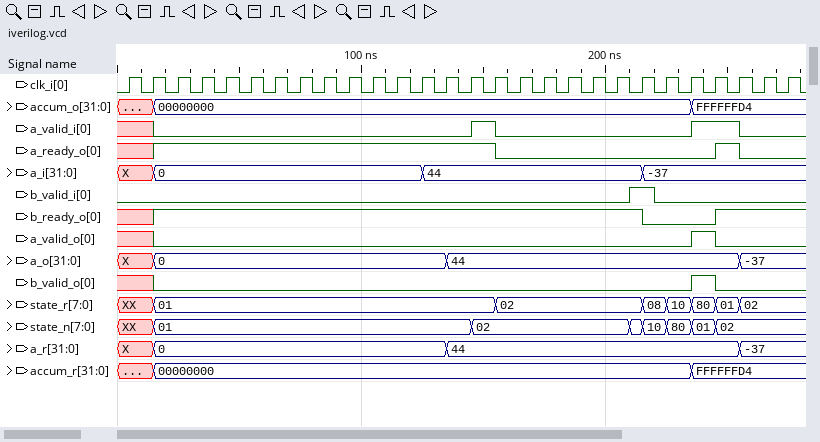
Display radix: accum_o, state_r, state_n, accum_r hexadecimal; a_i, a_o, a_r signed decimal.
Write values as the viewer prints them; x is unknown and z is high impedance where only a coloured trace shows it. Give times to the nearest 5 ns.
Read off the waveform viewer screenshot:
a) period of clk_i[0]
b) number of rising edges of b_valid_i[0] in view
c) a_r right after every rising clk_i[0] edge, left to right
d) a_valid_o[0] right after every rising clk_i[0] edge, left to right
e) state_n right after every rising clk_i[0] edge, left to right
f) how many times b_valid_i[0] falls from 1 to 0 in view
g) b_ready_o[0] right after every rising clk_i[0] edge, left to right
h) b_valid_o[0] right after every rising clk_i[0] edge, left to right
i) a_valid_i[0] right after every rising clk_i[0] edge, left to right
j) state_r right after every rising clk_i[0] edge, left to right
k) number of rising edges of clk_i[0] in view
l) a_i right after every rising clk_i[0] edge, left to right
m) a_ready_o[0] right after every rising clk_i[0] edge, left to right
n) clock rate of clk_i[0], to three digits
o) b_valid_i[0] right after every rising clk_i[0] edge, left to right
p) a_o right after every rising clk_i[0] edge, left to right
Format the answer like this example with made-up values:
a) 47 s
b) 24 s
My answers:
a) 10 ns
b) 1
c) X, 0, 0, 0, 0, 0, 0, 0, 0, 0, 0, 0, 0, 44, 44, 44, 44, 44, 44, 44, 44, 44, 44, 44, 44, -37, -37, -37
d) x 0 0 0 0 0 0 0 0 0 0 0 0 0 0 0 0 0 0 0 0 0 0 1 0 0 0 0
e) XX, 01, 01, 01, 01, 01, 01, 01, 01, 01, 01, 01, 01, 01, 02, 02, 02, 02, 02, 02, 02, 10, 80, 01, 02, 02, 02, 02
f) 1
g) x 1 1 1 1 1 1 1 1 1 1 1 1 1 1 1 1 1 1 1 1 0 0 0 1 1 1 1
h) x 0 0 0 0 0 0 0 0 0 0 0 0 0 0 0 0 0 0 0 0 0 0 1 0 0 0 0
i) x 0 0 0 0 0 0 0 0 0 0 0 0 0 1 0 0 0 0 0 0 0 0 1 1 0 0 0
j) XX, 01, 01, 01, 01, 01, 01, 01, 01, 01, 01, 01, 01, 01, 01, 02, 02, 02, 02, 02, 02, 08, 10, 80, 01, 02, 02, 02
k) 28
l) X, 0, 0, 0, 0, 0, 0, 0, 0, 0, 0, 0, 44, 44, 44, 44, 44, 44, 44, 44, 44, -37, -37, -37, -37, -37, -37, -37
m) x 1 1 1 1 1 1 1 1 1 1 1 1 1 1 0 0 0 0 0 0 0 0 0 1 0 0 0
n) 100 MHz
o) 0 0 0 0 0 0 0 0 0 0 0 0 0 0 0 0 0 0 0 0 0 1 0 0 0 0 0 0
p) X, 0, 0, 0, 0, 0, 0, 0, 0, 0, 0, 0, 0, 44, 44, 44, 44, 44, 44, 44, 44, 44, 44, 44, 44, -37, -37, -37
